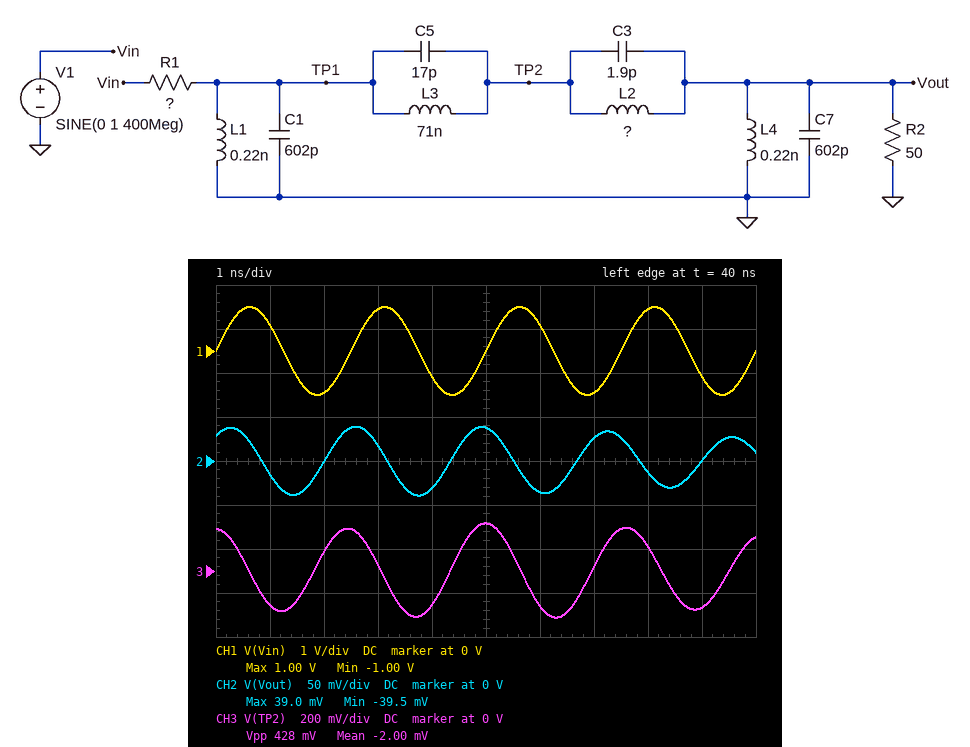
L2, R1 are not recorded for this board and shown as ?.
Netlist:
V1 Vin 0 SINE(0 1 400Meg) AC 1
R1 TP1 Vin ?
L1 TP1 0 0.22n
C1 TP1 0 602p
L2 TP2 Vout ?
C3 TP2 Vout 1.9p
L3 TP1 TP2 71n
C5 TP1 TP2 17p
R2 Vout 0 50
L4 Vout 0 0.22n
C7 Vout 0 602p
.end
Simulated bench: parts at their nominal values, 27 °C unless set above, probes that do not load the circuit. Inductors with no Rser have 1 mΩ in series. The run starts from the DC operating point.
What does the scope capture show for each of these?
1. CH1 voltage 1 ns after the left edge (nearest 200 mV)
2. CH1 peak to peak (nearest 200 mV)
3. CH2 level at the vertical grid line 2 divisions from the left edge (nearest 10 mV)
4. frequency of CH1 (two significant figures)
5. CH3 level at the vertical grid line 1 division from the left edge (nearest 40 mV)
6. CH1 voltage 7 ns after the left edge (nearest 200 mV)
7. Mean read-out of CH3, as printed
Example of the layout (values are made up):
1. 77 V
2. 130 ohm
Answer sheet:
1. 600 mV
2. 2.0 V
3. 0 V
4. 400 MHz
5. -160 mV
6. -1.0 V
7. -2.00 mV
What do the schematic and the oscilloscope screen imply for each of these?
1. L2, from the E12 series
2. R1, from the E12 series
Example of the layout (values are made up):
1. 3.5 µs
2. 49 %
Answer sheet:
1. 18 nH
2. 27 Ω
